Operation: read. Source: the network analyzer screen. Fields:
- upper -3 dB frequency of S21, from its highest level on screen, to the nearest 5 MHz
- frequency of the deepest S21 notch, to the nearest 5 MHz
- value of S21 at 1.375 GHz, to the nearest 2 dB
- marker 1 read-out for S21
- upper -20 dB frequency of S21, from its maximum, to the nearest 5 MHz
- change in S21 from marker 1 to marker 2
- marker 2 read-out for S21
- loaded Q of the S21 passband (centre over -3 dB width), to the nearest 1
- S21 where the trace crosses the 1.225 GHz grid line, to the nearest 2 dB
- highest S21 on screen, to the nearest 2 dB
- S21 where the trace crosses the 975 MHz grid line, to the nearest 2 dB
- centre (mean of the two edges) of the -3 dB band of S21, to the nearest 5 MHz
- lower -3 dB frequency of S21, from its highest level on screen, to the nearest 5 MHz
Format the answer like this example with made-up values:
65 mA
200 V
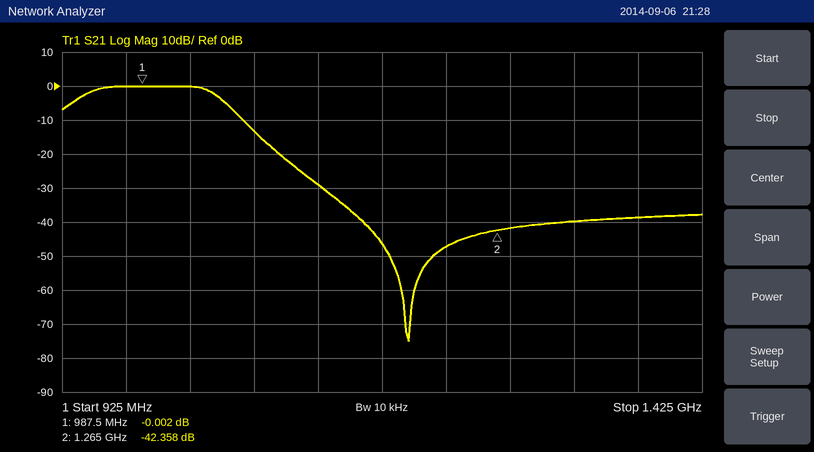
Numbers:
1.045 GHz
1.195 GHz
-38 dB
-0.002 dB
1.095 GHz
-42.356 dB
-42.358 dB
9
-48 dB
0 dB
0 dB
995 MHz
940 MHz
